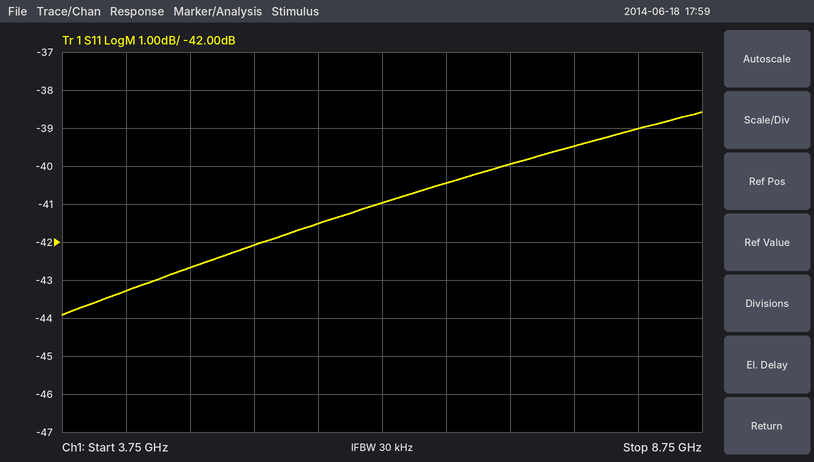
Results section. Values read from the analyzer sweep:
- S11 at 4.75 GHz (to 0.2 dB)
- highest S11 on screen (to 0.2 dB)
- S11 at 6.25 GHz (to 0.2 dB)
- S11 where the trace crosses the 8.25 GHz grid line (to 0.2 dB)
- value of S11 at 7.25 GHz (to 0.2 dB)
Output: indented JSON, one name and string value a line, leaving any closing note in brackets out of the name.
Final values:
{
  "S11 at 4.75 GHz": "-42.6 dB",
  "highest S11 on screen": "-38.6 dB",
  "S11 at 6.25 GHz": "-41.0 dB",
  "S11 where the trace crosses the 8.25 GHz grid line": "-39.0 dB",
  "value of S11 at 7.25 GHz": "-40.0 dB"
}
